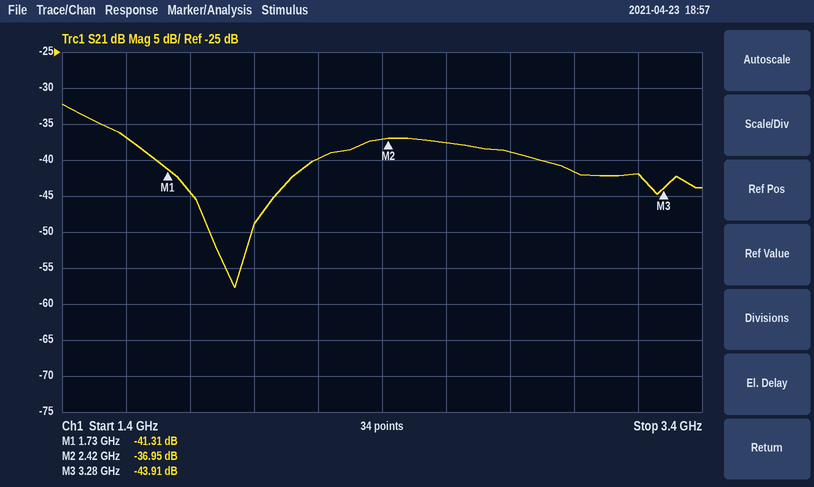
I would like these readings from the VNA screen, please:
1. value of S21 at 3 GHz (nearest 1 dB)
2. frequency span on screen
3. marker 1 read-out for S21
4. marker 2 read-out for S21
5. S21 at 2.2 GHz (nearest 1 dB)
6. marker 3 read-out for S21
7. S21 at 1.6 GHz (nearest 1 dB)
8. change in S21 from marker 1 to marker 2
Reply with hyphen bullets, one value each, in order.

- -42 dB
- 2 GHz
- -41.31 dB
- -36.95 dB
- -40 dB
- -43.91 dB
- -37 dB
- 4.36 dB
